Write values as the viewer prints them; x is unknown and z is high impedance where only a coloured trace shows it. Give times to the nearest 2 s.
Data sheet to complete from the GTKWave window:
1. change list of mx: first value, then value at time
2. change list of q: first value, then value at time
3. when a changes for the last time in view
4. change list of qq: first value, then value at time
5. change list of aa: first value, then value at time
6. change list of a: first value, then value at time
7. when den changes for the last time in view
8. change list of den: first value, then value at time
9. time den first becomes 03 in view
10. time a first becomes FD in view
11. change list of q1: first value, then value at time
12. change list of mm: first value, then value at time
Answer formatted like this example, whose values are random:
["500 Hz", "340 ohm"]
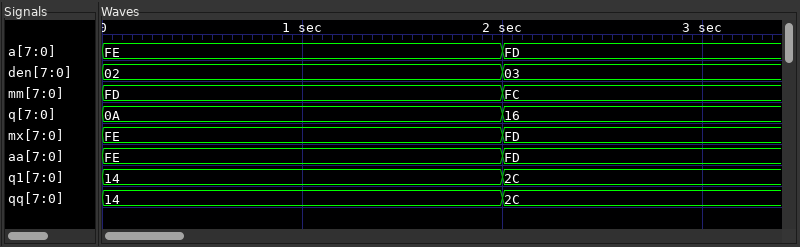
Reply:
["FE, FD at 2 s", "0A, 16 at 2 s", "2 s", "14, 2C at 2 s", "FE, FD at 2 s", "FE, FD at 2 s", "2 s", "02, 03 at 2 s", "2 s", "2 s", "14, 2C at 2 s", "FD, FC at 2 s"]
